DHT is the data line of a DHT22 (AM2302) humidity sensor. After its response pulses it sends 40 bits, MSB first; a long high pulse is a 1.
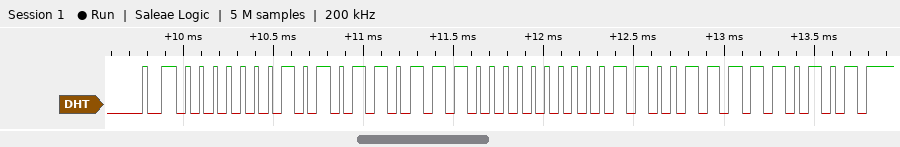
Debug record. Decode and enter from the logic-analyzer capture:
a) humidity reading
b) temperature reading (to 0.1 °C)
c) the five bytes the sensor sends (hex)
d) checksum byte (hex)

34.7 %
-2.5 °C
01 5B 80 19 F5
0xF5
